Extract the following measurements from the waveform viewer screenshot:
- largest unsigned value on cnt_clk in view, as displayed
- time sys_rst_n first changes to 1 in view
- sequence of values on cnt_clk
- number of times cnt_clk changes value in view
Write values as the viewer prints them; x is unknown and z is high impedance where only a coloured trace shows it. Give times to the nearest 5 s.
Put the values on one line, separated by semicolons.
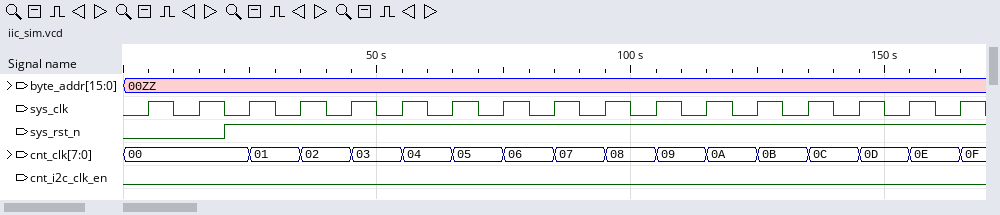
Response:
0F; 20 s; 00, 01, 02, 03, 04, 05, 06, 07, 08, 09, 0A, 0B, 0C, 0D, 0E, 0F; 15
